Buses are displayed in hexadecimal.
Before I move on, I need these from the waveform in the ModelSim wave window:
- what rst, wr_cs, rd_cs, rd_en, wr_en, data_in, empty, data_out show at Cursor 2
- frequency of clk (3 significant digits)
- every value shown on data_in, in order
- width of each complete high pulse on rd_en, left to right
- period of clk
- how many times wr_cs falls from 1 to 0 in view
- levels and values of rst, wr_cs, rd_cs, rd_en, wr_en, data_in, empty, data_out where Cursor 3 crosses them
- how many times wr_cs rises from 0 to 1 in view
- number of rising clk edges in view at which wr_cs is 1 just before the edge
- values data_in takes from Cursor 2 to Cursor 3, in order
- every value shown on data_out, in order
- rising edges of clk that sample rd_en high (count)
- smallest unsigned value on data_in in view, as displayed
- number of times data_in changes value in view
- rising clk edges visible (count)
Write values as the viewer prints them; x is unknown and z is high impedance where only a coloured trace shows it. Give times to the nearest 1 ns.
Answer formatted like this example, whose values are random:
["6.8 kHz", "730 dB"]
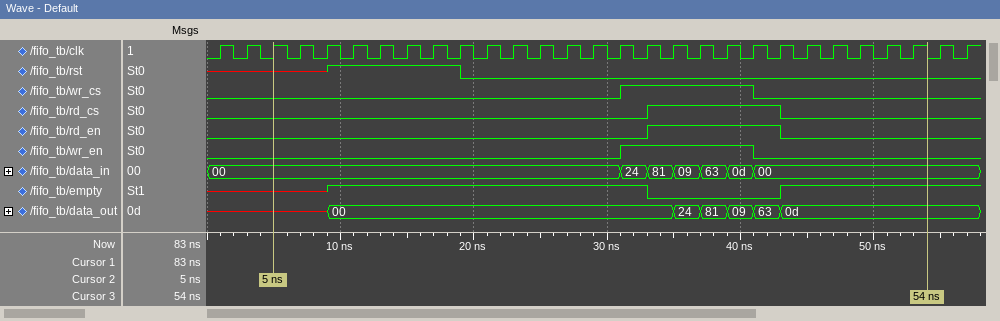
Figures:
["rst=x, wr_cs=0, rd_cs=0, rd_en=0, wr_en=0, data_in=00, empty=x, data_out=x", "500 MHz", "00, 24, 81, 09, 63, 0d, 00", "10 ns", "2 ns", "1", "rst=0, wr_cs=0, rd_cs=0, rd_en=0, wr_en=0, data_in=00, empty=1, data_out=0d", "1", "5", "00, 24, 81, 09, 63, 0d, 00", "x, 00, 24, 81, 09, 63, 0d", "5", "00", "6", "29"]
